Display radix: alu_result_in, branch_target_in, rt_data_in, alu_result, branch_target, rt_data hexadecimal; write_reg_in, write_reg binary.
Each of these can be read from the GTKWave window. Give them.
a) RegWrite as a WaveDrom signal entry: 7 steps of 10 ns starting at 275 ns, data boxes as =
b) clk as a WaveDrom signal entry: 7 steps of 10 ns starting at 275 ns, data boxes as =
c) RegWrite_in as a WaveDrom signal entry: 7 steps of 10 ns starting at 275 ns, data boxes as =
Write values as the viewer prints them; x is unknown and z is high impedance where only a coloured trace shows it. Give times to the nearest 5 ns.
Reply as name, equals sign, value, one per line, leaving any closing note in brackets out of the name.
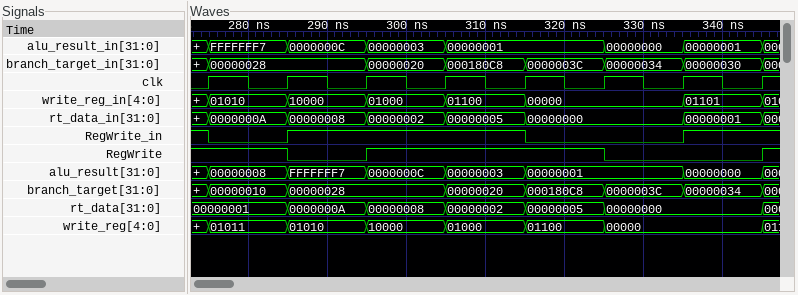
RegWrite as a WaveDrom signal entry: 7 steps of 10 ns starting at 275 ns, data boxes as = = {name: 'RegWrite', wave: '101..0.'}
clk as a WaveDrom signal entry: 7 steps of 10 ns starting at 275 ns, data boxes as = = {name: 'clk', wave: 'p......'}
RegWrite_in as a WaveDrom signal entry: 7 steps of 10 ns starting at 275 ns, data boxes as = = {name: 'RegWrite_in', wave: '01..0.1'}
